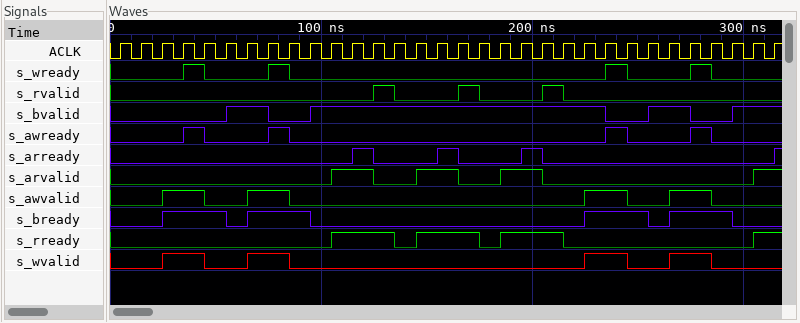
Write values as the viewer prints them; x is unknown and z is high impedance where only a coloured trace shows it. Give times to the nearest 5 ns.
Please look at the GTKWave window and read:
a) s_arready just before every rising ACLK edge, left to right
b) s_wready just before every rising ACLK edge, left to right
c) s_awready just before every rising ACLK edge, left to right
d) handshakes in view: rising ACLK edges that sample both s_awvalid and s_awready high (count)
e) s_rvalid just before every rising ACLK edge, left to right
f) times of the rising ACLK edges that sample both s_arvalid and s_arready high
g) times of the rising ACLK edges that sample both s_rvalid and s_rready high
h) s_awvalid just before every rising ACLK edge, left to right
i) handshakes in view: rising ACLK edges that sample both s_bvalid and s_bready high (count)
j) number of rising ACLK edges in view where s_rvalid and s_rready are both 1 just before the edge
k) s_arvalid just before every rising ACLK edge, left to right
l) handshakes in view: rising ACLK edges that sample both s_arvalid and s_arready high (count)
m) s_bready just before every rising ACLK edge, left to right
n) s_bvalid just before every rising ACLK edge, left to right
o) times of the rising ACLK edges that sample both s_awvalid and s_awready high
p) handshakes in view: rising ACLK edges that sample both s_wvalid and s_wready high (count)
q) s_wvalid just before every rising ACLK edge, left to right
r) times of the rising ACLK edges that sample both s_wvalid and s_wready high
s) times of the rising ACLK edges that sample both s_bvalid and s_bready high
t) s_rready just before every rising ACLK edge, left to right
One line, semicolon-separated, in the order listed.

0 0 0 0 0 0 0 0 0 0 0 0 1 0 0 0 1 0 0 0 1 0 0 0 0 0 0 0 0 0 0 0; 0 0 0 0 1 0 0 0 1 0 0 0 0 0 0 0 0 0 0 0 0 0 0 0 1 0 0 0 1 0 0 0; 0 0 0 0 1 0 0 0 1 0 0 0 0 0 0 0 0 0 0 0 0 0 0 0 1 0 0 0 1 0 0 0; 4; 0 0 0 0 0 0 0 0 0 0 0 0 0 1 0 0 0 1 0 0 0 1 0 0 0 0 0 0 0 0 0 0; 125 ns, 165 ns, 205 ns; 135 ns, 175 ns, 215 ns; 0 0 0 1 1 0 0 1 1 0 0 0 0 0 0 0 0 0 0 0 0 0 0 1 1 0 0 1 1 0 0 0; 3; 3; 0 0 0 0 0 0 0 0 0 0 0 1 1 0 0 1 1 0 0 1 1 0 0 0 0 0 0 0 0 0 0 1; 3; 0 0 0 1 1 1 0 1 1 1 0 0 0 0 0 0 0 0 0 0 0 0 0 1 1 1 0 1 1 1 0 0; 0 0 0 0 0 0 1 1 0 0 1 1 1 1 1 1 1 1 1 1 1 1 1 1 0 0 1 1 0 0 1 1; 45 ns, 85 ns, 245 ns, 285 ns; 4; 0 0 0 1 1 0 0 1 1 0 0 0 0 0 0 0 0 0 0 0 0 0 0 1 1 0 0 1 1 0 0 0; 45 ns, 85 ns, 245 ns, 285 ns; 75 ns, 235 ns, 275 ns; 0 0 0 0 0 0 0 0 0 0 0 1 1 1 0 1 1 1 0 1 1 1 0 0 0 0 0 0 0 0 0 1
